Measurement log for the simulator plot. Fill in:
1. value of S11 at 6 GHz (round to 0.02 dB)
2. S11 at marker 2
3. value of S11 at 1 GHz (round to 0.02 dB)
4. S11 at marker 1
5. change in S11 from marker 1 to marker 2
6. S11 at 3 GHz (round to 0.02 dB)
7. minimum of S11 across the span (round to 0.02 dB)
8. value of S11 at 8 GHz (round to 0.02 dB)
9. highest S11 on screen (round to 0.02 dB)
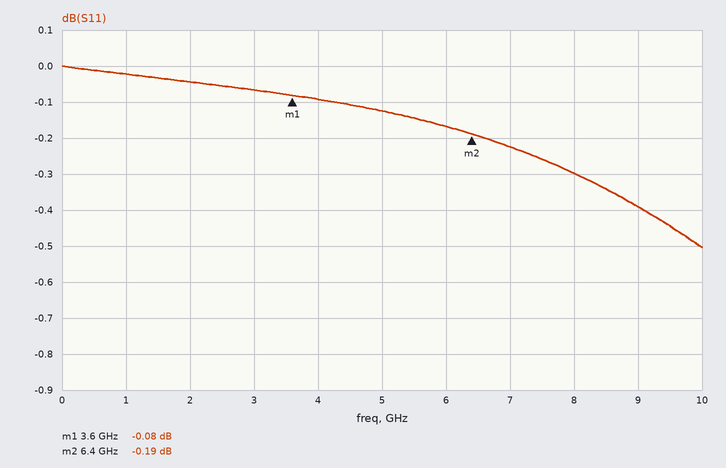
-0.16 dB
-0.19 dB
-0.02 dB
-0.08 dB
-0.11 dB
-0.06 dB
-0.50 dB
-0.30 dB
0.00 dB
